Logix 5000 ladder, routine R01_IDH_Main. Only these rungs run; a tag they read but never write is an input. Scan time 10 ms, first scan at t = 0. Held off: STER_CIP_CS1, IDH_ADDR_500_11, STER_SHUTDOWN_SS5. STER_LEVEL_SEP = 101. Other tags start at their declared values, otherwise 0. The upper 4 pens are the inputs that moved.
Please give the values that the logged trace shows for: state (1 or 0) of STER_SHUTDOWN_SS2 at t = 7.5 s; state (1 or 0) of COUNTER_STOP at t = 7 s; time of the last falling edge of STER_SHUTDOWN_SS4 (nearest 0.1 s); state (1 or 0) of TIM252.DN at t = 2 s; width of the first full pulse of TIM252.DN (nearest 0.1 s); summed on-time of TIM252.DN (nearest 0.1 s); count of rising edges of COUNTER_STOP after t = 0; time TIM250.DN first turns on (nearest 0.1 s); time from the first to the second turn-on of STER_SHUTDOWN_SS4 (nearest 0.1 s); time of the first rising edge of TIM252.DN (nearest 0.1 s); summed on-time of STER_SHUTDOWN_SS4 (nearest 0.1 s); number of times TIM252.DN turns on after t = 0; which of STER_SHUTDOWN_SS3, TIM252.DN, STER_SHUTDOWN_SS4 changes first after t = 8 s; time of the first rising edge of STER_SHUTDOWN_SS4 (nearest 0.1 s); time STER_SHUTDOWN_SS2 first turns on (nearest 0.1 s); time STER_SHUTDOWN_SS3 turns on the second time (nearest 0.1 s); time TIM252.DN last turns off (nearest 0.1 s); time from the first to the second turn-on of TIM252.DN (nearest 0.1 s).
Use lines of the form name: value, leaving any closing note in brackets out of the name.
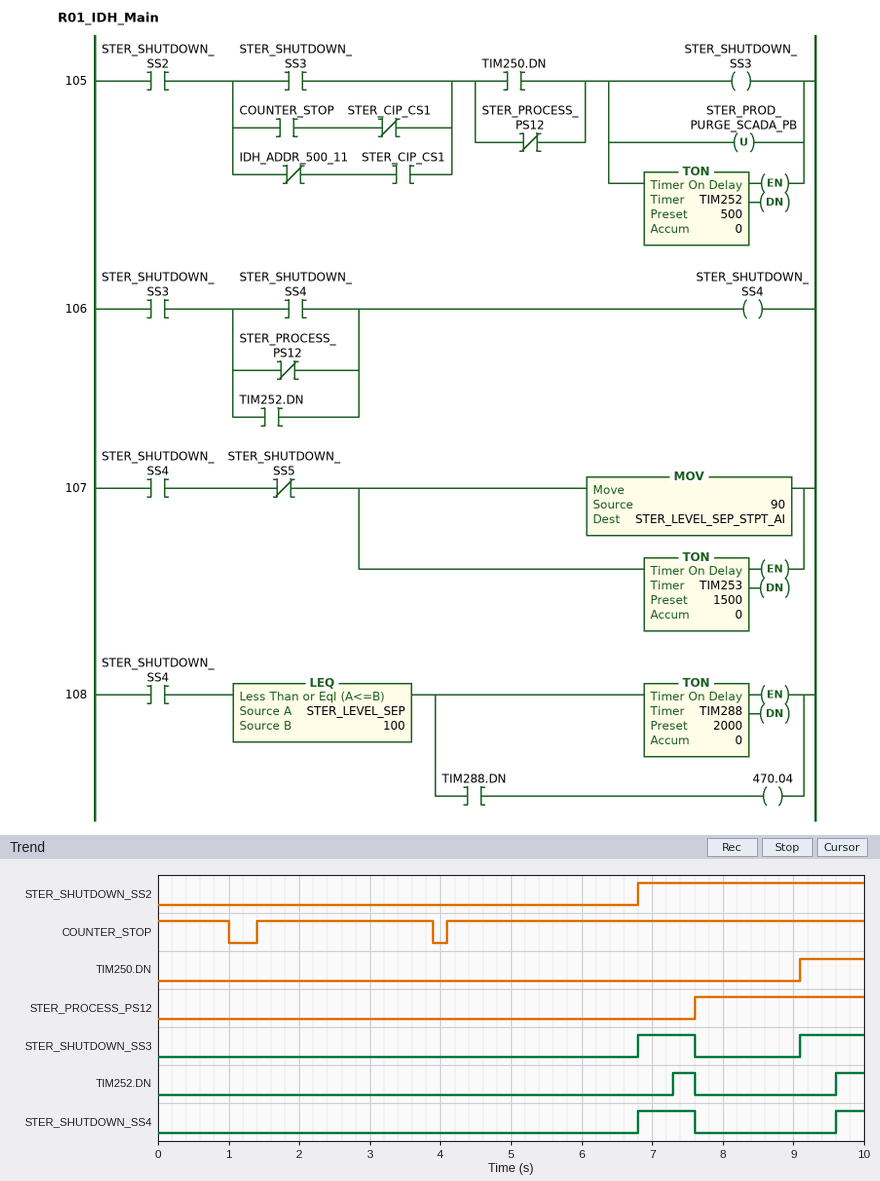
state (1 or 0) of STER_SHUTDOWN_SS2 at t = 7.5 s: 1
state (1 or 0) of COUNTER_STOP at t = 7 s: 1
time of the last falling edge of STER_SHUTDOWN_SS4: 7.6 s
state (1 or 0) of TIM252.DN at t = 2 s: 0
width of the first full pulse of TIM252.DN: 0.3 s
summed on-time of TIM252.DN: 0.7 s
count of rising edges of COUNTER_STOP after t = 0: 2
time TIM250.DN first turns on: 9.1 s
time from the first to the second turn-on of STER_SHUTDOWN_SS4: 2.8 s
time of the first rising edge of TIM252.DN: 7.3 s
summed on-time of STER_SHUTDOWN_SS4: 1.2 s
number of times TIM252.DN turns on after t = 0: 2
which of STER_SHUTDOWN_SS3, TIM252.DN, STER_SHUTDOWN_SS4 changes first after t = 8 s: STER_SHUTDOWN_SS3
time of the first rising edge of STER_SHUTDOWN_SS4: 6.8 s
time STER_SHUTDOWN_SS2 first turns on: 6.8 s
time STER_SHUTDOWN_SS3 turns on the second time: 9.1 s
time TIM252.DN last turns off: 7.6 s
time from the first to the second turn-on of TIM252.DN: 2.3 s
